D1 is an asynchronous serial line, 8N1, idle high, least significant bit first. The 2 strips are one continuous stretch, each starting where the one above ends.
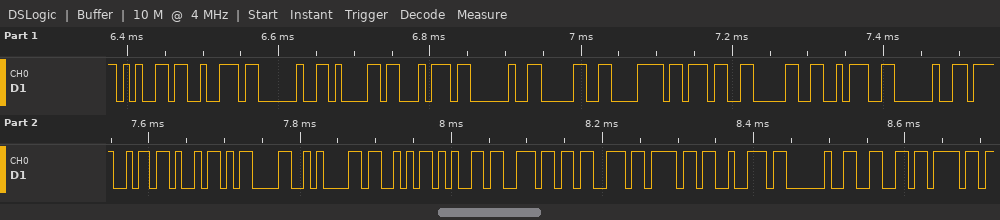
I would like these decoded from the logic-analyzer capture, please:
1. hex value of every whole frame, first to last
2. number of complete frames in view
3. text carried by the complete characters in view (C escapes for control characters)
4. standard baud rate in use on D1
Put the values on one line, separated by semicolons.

0x65 0x72 0x20 0x61 0x74 0x20 0x30 0x78 0x37 0x30 0x3A 0x20 0x4F 0x4B 0x0D 0x0A 0x53 0x65 0x6E 0x73 0x6F 0x72 0x20 0x66 0x6F; 25; "er at 0x70: OK\r\nSensor fo"; 115200 baud
